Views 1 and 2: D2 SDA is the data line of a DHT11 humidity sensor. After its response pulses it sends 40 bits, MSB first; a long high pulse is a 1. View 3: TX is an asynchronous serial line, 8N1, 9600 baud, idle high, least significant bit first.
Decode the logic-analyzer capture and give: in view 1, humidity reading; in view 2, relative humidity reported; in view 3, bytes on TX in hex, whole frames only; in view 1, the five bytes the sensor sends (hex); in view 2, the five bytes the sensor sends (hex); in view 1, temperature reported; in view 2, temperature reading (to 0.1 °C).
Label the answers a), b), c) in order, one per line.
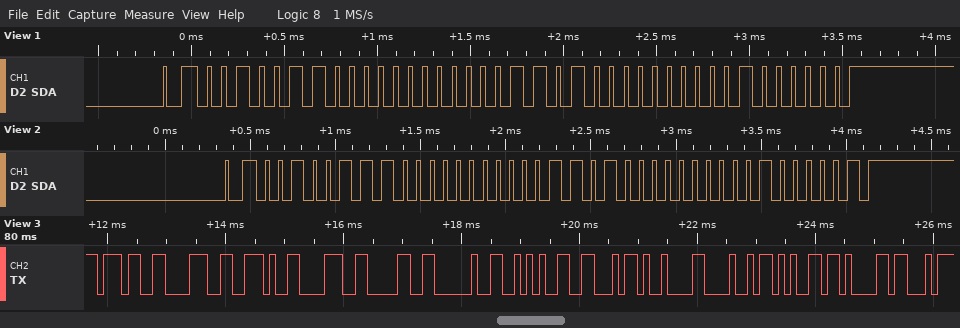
a) 38 %
b) 39 %
c) 37 38 2E 38 30 20 2A 46 09 48 65 61
d) 26 00 1A 00 40
e) 27 00 1A 00 41
f) 26.0 °C
g) 26.0 °C
